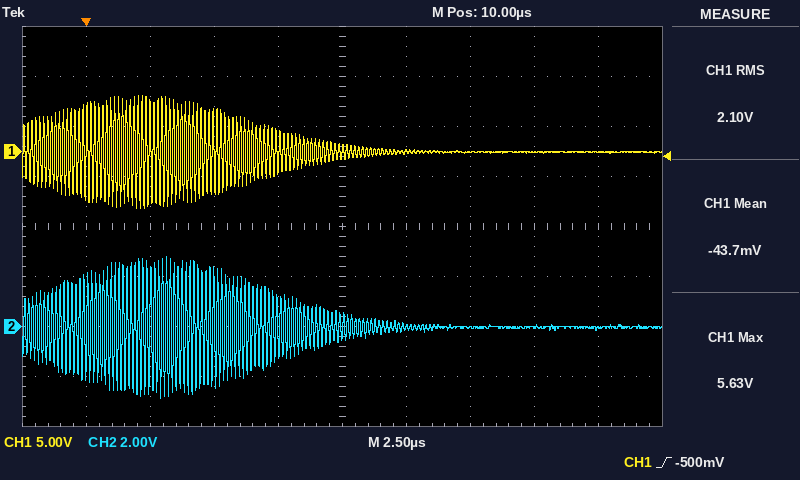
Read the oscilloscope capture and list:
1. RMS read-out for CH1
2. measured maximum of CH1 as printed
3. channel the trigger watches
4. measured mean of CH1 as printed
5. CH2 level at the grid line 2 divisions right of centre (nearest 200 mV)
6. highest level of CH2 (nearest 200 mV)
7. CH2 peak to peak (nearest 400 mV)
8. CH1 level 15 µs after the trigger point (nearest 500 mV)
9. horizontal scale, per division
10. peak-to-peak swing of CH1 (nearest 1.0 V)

2.10 V
5.63 V
CH1
-43.7 mV
0.0 V
2.8 V
5.6 V
0.0 V
2.5 µs
11.0 V
